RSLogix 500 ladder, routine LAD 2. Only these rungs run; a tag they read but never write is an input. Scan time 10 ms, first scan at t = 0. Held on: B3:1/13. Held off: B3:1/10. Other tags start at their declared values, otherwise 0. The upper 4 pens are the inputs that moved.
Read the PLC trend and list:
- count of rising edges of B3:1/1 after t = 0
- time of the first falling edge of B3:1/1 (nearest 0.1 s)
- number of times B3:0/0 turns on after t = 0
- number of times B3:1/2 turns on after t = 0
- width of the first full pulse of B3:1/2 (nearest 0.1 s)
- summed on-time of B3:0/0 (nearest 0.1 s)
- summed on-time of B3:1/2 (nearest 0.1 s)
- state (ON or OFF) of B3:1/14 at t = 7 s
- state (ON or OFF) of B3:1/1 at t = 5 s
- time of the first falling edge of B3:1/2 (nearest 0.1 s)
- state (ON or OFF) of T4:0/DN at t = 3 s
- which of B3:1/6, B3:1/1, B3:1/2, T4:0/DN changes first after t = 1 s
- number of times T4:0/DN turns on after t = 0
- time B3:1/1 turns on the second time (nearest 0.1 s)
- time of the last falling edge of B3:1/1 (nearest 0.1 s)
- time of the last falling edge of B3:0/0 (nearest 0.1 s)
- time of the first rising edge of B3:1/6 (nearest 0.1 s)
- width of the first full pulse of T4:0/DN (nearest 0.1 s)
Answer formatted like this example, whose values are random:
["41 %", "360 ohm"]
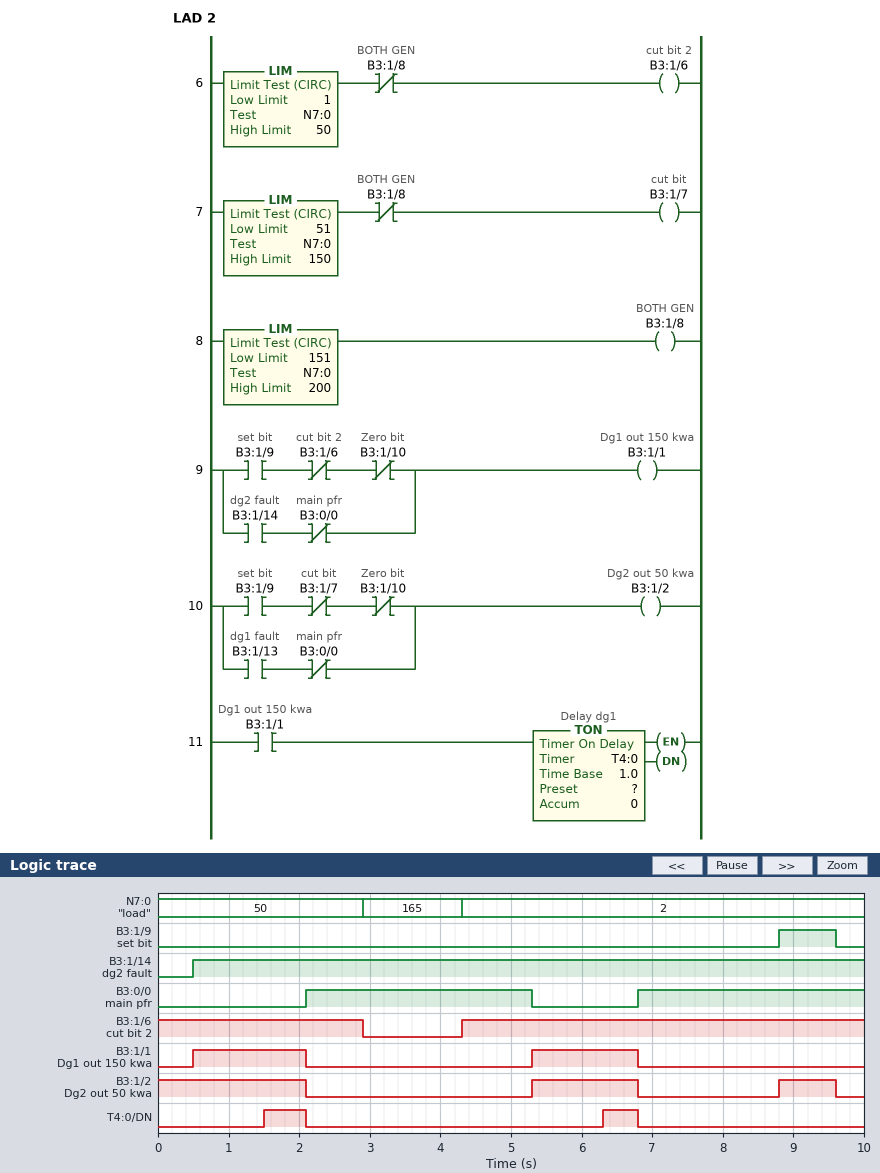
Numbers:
["2", "2.1 s", "2", "2", "1.5 s", "6.4 s", "4.4 s", "ON", "OFF", "2.1 s", "OFF", "T4:0/DN", "2", "5.3 s", "6.8 s", "5.3 s", "4.3 s", "0.6 s"]
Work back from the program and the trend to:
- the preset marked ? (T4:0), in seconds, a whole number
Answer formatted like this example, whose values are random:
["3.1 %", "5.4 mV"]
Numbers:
["1 s"]
